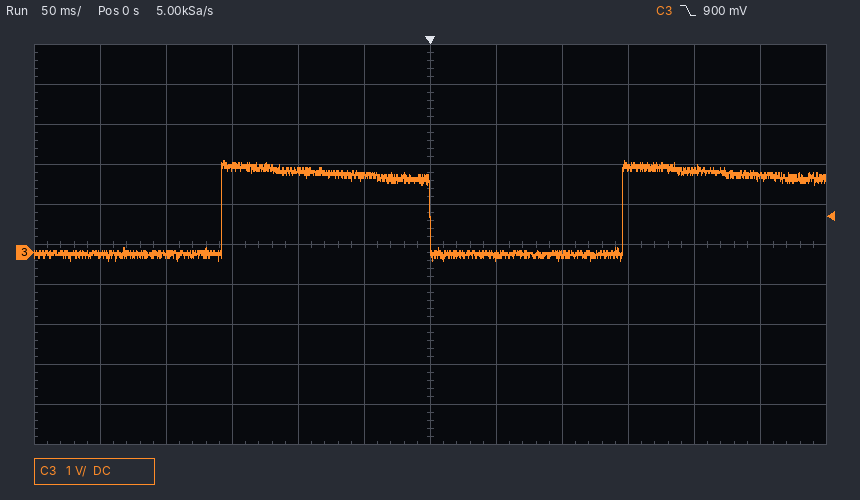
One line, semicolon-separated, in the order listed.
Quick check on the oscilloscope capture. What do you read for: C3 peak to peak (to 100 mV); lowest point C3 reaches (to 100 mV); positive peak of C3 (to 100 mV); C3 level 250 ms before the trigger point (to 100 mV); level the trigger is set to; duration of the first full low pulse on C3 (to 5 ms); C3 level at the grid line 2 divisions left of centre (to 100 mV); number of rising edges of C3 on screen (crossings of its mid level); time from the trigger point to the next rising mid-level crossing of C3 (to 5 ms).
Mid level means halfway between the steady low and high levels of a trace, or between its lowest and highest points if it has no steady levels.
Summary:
2.5 V; -200 mV; 2.3 V; 0.0 V; 900 mV; 145 ms; 2.0 V; 2; 145 ms
